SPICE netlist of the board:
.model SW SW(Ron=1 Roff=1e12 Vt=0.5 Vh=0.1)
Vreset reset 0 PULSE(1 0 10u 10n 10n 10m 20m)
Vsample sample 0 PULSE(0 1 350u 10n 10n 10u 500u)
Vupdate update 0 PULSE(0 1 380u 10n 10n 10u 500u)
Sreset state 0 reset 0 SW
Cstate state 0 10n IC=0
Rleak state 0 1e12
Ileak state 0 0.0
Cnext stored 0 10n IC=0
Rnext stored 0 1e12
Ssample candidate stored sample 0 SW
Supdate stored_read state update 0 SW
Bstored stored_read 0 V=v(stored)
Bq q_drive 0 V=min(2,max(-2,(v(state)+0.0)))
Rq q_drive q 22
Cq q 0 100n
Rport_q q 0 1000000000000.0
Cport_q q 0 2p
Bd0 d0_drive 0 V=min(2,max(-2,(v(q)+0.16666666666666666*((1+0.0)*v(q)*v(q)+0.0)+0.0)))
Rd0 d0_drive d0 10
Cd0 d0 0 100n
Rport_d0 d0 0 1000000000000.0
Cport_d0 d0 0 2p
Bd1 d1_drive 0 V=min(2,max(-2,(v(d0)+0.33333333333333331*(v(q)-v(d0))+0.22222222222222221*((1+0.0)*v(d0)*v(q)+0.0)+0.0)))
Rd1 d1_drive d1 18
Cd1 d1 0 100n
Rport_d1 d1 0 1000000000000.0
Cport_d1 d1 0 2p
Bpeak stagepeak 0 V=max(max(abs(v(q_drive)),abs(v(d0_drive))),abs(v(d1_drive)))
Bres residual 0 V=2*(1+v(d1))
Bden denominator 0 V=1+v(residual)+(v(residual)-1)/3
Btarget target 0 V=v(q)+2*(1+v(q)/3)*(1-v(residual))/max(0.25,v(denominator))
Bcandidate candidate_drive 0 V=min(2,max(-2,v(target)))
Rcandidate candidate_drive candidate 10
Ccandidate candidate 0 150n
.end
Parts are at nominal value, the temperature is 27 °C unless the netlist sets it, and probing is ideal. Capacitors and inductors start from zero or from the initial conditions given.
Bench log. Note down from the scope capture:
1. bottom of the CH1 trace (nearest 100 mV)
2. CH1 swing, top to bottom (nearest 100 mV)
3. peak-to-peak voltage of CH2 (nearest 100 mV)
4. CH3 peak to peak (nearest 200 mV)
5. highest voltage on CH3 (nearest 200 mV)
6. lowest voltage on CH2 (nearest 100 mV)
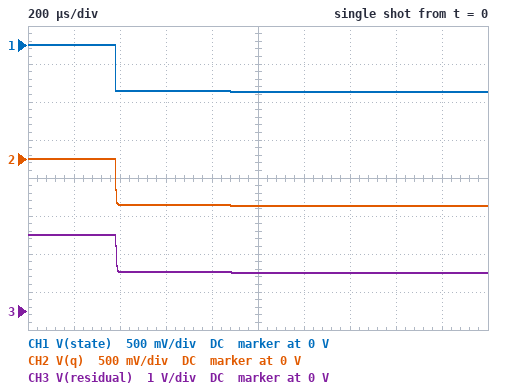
-600 mV
600 mV
600 mV
1.0 V
2.0 V
-600 mV
